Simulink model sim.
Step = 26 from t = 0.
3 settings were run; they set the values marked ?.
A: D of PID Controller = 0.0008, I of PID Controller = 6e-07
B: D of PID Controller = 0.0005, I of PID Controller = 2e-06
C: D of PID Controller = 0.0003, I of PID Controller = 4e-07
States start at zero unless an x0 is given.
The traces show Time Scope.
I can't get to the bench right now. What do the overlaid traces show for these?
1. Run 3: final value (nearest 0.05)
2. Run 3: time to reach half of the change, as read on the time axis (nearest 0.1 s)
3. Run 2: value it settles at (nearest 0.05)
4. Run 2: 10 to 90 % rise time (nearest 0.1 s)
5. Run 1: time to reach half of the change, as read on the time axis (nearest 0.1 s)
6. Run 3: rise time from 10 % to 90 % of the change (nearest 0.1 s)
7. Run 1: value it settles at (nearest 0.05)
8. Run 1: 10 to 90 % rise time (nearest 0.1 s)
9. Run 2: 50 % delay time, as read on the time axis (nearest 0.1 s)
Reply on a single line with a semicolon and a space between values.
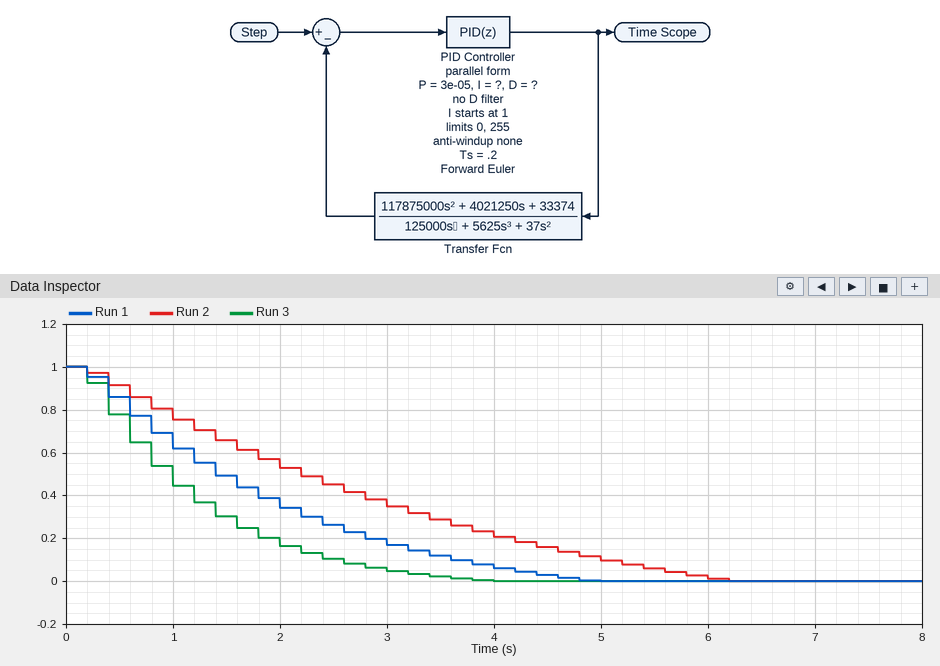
0.00; 1.0 s; 0.00; 4.4 s; 1.4 s; 2.2 s; 0.00; 3.2 s; 2.2 s
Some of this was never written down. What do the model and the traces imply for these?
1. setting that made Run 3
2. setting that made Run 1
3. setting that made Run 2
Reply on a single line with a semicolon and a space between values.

A; B; C
